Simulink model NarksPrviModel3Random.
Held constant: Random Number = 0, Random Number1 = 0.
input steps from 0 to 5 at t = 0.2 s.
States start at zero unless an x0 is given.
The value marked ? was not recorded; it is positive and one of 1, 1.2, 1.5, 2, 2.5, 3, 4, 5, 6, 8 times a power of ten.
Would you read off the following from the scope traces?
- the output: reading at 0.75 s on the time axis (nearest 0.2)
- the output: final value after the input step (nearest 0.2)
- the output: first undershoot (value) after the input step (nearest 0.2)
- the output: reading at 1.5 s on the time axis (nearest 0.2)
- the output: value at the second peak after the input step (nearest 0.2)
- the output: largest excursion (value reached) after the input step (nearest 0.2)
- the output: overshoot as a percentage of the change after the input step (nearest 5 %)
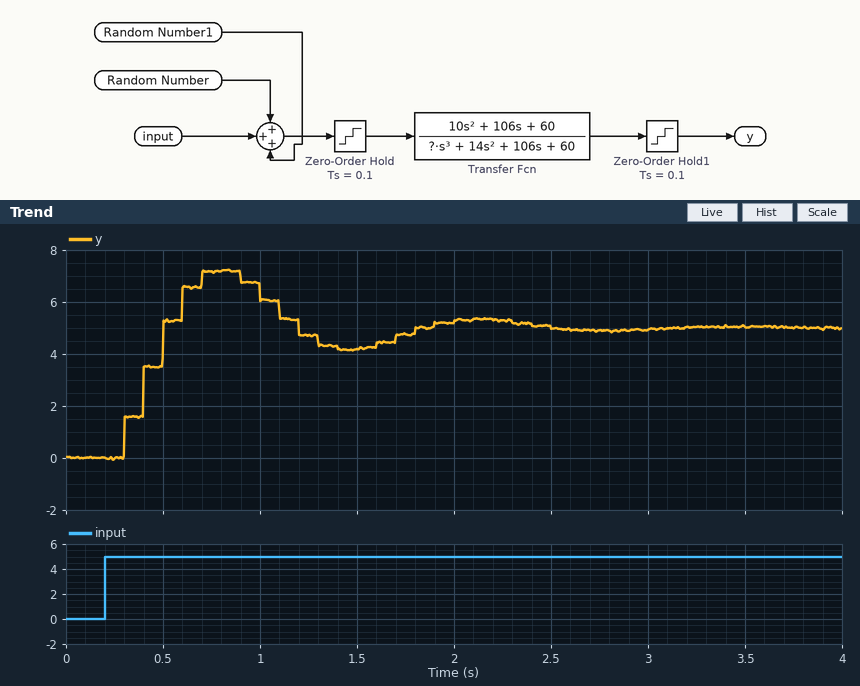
7.2
5.0
4.2
4.2
5.4
7.2
45 %
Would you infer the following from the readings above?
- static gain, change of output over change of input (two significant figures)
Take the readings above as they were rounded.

1.0
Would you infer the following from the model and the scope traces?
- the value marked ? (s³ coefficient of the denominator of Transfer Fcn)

4
